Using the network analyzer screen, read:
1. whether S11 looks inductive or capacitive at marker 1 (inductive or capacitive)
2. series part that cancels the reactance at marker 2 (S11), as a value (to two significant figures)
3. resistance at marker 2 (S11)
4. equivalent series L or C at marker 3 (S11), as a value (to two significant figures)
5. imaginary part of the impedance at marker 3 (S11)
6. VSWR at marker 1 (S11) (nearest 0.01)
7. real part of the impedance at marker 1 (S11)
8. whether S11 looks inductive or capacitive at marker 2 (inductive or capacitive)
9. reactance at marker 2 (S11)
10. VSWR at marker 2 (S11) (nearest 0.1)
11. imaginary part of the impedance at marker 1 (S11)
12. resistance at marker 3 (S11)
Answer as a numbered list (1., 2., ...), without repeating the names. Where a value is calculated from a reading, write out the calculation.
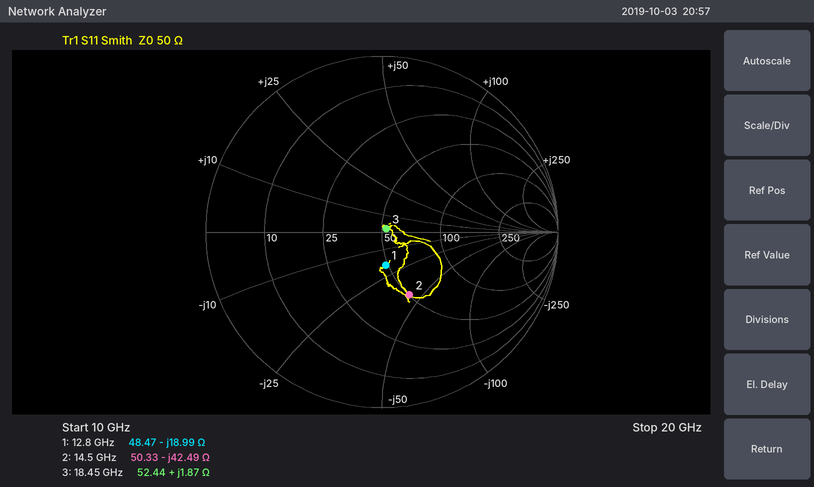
1. capacitive
2. L = 42.49 Ω/(2π × 14.5 GHz) ≈ 466 pH, so 470 pH to two significant figures
3. 50.33 Ω
4. L = 1.87 Ω/(2π × 18.45 GHz) ≈ 16 pH
5. +1.87 Ω
6. 1.47
7. 48.47 Ω
8. capacitive
9. -42.49 Ω
10. 2.3
11. -18.99 Ω
12. 52.44 Ω
